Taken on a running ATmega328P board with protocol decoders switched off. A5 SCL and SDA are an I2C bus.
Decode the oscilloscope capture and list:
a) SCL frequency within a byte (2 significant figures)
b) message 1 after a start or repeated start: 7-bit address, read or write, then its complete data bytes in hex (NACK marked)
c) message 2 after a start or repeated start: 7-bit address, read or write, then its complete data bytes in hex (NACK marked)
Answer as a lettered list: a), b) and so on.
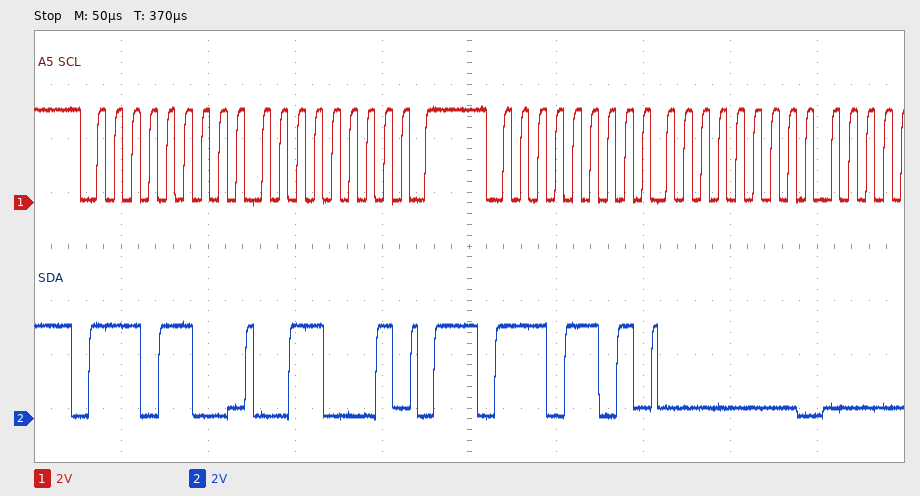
a) 100 kHz
b) 0x76 write: 31
c) 0x76 read: 00
